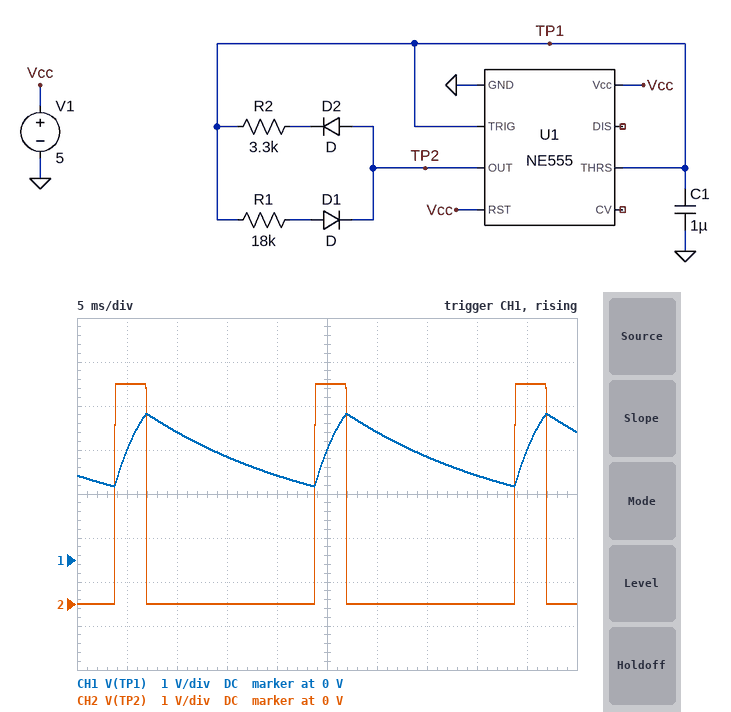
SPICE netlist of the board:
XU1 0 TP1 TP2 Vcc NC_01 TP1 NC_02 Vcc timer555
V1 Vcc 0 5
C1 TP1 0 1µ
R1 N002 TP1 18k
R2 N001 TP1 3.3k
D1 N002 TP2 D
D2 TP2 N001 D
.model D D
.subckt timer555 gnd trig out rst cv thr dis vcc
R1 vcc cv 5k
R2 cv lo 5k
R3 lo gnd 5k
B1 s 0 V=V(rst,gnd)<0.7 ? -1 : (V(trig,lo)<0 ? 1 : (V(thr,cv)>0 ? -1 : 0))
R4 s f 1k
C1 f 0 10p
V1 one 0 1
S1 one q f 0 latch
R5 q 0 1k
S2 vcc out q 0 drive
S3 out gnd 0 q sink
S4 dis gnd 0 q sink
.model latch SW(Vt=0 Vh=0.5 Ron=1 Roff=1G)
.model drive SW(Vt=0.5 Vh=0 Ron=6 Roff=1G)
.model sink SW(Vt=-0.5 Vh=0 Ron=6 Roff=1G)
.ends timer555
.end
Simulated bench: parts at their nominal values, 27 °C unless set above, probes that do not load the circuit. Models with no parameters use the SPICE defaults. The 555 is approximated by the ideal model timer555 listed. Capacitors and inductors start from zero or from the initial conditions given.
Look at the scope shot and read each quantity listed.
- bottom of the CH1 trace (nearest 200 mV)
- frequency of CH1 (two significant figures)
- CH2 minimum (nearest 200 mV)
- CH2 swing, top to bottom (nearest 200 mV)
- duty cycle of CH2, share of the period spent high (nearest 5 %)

1.6 V
50 Hz
0 V
5.0 V
15 %
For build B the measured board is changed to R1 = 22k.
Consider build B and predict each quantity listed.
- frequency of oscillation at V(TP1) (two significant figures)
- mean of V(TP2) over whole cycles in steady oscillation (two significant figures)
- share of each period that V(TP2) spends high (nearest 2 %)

42 Hz
670 mV
14 %
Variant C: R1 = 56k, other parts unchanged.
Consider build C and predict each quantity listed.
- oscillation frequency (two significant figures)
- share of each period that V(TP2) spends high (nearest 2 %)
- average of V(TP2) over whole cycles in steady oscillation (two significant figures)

18 Hz
6 %
290 mV
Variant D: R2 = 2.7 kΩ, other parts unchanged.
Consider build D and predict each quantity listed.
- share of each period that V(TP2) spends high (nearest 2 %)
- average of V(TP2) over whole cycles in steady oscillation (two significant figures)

14 %
670 mV
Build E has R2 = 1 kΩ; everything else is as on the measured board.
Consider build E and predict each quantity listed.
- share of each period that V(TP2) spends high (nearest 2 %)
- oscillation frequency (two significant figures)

6 %
56 Hz
